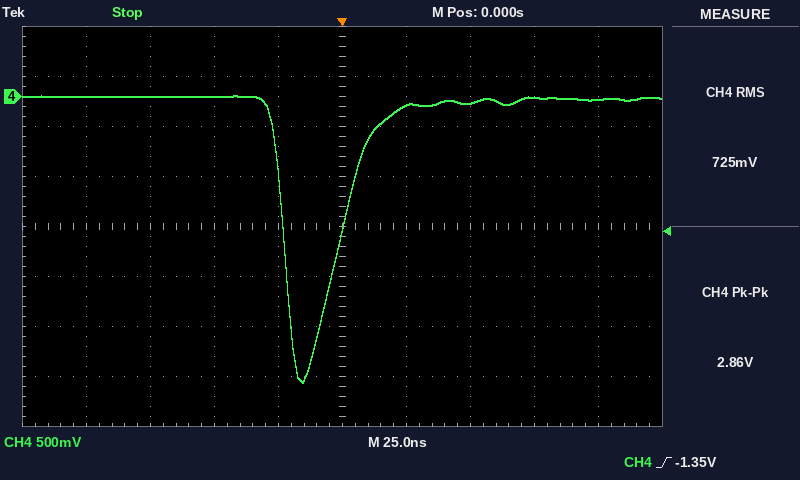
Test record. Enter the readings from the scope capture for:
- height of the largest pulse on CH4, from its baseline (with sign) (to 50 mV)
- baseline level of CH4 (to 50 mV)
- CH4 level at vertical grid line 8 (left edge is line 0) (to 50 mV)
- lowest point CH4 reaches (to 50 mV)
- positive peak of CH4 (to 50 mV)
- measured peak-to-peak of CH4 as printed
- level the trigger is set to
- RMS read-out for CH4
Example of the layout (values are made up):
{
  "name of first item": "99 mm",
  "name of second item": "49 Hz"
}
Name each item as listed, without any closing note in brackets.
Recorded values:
{
  "height of the largest pulse on CH4, from its baseline (with sign)": "-2.85 V",
  "baseline level of CH4": "0 mV",
  "CH4 level at vertical grid line 8 (left edge is line 0)": "0 mV",
  "lowest point CH4 reaches": "-2.85 V",
  "positive peak of CH4": "0 mV",
  "measured peak-to-peak of CH4 as printed": "2.86 V",
  "level the trigger is set to": "-1.35 V",
  "RMS read-out for CH4": "725 mV"
}
